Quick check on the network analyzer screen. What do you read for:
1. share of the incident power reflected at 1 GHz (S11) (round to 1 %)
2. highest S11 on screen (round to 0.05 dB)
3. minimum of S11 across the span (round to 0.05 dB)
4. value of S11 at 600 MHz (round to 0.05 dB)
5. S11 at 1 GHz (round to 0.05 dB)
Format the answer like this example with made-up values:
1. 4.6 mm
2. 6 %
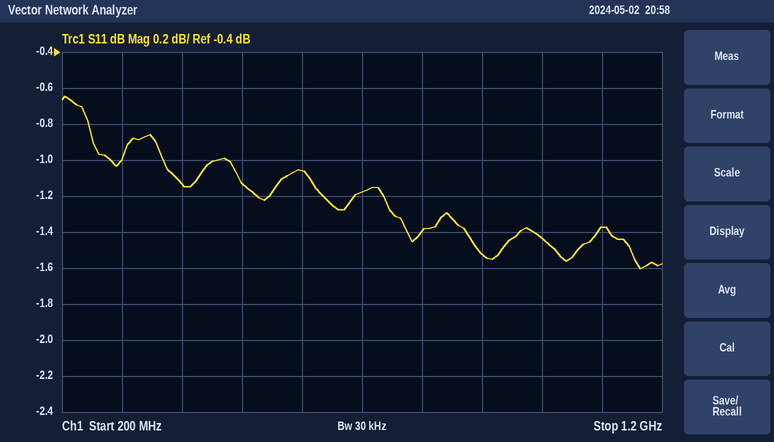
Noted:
1. 72 %
2. -0.65 dB
3. -1.60 dB
4. -1.05 dB
5. -1.45 dB
